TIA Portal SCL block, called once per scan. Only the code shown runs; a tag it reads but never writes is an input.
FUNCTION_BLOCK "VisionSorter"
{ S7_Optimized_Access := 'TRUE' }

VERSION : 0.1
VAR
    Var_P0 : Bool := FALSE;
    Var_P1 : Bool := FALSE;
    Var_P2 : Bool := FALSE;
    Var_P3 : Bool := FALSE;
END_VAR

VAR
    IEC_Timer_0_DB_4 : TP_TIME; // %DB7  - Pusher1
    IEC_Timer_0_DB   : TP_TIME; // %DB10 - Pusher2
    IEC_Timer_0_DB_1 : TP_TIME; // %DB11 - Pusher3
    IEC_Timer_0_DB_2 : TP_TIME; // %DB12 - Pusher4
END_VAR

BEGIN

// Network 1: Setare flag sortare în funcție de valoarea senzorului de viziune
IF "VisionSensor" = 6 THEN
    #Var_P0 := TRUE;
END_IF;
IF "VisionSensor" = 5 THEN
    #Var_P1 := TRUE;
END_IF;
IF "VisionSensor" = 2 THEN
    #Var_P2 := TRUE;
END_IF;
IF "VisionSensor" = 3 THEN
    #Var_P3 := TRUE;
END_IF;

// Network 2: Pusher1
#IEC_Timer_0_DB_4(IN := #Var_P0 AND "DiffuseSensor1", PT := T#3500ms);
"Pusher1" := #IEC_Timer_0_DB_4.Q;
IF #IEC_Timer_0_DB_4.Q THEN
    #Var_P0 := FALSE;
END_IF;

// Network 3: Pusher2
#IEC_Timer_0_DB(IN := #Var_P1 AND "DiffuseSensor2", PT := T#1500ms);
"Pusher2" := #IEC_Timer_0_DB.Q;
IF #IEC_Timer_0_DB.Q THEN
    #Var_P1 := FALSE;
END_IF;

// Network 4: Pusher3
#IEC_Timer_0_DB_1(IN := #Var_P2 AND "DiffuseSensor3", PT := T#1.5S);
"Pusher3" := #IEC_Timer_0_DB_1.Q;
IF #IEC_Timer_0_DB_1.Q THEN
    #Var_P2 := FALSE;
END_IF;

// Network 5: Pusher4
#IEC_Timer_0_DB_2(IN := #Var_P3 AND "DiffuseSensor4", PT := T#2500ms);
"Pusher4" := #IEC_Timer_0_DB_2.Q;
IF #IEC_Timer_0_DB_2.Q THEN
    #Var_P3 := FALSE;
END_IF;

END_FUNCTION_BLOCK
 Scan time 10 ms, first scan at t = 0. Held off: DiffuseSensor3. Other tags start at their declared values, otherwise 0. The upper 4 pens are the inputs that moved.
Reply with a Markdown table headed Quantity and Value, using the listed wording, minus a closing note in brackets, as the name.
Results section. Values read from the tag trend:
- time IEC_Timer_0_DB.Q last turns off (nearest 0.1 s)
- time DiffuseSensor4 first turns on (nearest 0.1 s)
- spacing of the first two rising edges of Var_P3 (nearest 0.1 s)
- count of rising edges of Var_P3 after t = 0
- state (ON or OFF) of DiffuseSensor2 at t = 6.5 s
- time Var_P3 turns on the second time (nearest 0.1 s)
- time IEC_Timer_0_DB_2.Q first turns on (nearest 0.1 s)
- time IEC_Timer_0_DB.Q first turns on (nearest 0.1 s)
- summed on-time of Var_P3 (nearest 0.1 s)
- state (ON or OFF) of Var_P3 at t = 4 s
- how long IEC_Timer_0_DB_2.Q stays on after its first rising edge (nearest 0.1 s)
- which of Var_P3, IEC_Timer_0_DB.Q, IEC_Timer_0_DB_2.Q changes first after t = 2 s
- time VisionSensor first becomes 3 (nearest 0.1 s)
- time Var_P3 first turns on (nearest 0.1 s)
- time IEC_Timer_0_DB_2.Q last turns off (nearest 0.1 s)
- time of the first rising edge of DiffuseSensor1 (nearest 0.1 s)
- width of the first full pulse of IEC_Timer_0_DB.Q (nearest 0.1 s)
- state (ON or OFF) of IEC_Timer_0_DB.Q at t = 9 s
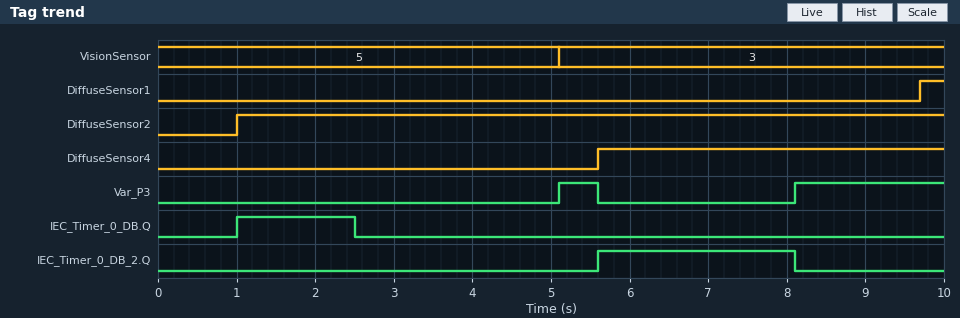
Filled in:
| Quantity | Value |
|---|---|
| time IEC_Timer_0_DB.Q last turns off | 2.5 s |
| time DiffuseSensor4 first turns on | 5.6 s |
| spacing of the first two rising edges of Var_P3 | 3.0 s |
| count of rising edges of Var_P3 after t = 0 | 2 |
| state (ON or OFF) of DiffuseSensor2 at t = 6.5 s | ON |
| time Var_P3 turns on the second time | 8.1 s |
| time IEC_Timer_0_DB_2.Q first turns on | 5.6 s |
| time IEC_Timer_0_DB.Q first turns on | 1.0 s |
| summed on-time of Var_P3 | 2.4 s |
| state (ON or OFF) of Var_P3 at t = 4 s | OFF |
| how long IEC_Timer_0_DB_2.Q stays on after its first rising edge | 2.5 s |
| which of Var_P3, IEC_Timer_0_DB.Q, IEC_Timer_0_DB_2.Q changes first after t = 2 s | IEC_Timer_0_DB.Q |
| time VisionSensor first becomes 3 | 5.1 s |
| time Var_P3 first turns on | 5.1 s |
| time IEC_Timer_0_DB_2.Q last turns off | 8.1 s |
| time of the first rising edge of DiffuseSensor1 | 9.7 s |
| width of the first full pulse of IEC_Timer_0_DB.Q | 1.5 s |
| state (ON or OFF) of IEC_Timer_0_DB.Q at t = 9 s | OFF |
